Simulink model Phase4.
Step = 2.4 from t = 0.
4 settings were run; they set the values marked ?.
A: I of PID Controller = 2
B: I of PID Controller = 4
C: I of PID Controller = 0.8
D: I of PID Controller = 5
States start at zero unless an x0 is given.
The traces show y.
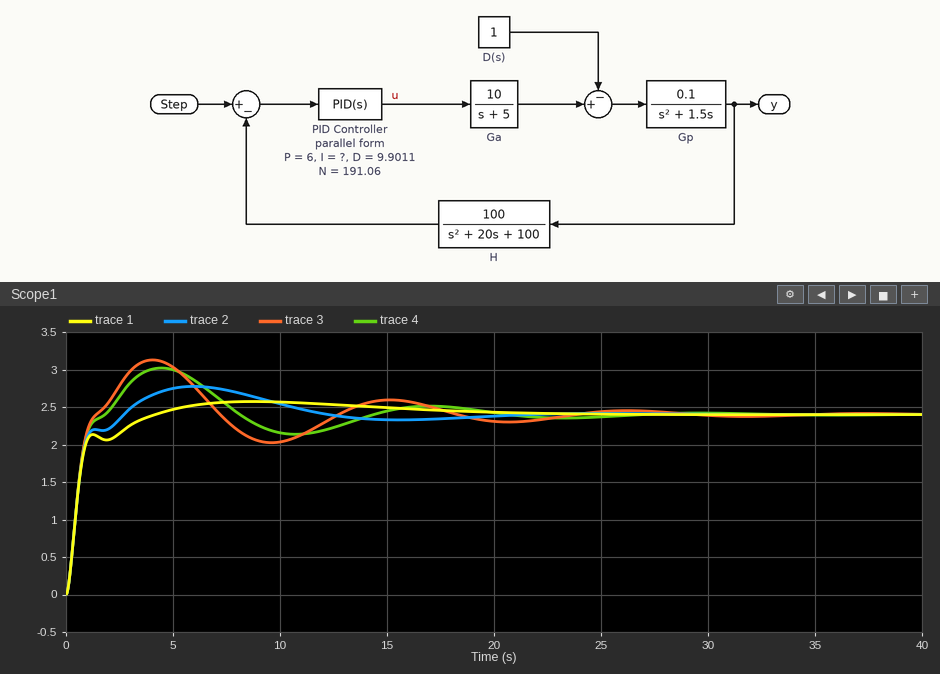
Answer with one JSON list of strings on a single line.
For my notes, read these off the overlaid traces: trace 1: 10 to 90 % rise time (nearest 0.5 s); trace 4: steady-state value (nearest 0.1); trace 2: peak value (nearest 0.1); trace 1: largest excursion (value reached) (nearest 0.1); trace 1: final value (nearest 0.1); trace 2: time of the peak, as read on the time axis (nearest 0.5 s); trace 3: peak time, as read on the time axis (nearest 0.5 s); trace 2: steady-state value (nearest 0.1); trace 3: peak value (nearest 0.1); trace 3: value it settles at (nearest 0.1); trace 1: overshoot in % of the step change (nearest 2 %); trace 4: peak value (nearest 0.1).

["2.5 s", "2.4", "2.8", "2.6", "2.4", "6.0 s", "4.0 s", "2.4", "3.1", "2.4", "8 %", "3.0"]
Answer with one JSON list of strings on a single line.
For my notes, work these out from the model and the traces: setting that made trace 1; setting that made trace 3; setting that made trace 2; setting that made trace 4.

["C", "D", "A", "B"]
